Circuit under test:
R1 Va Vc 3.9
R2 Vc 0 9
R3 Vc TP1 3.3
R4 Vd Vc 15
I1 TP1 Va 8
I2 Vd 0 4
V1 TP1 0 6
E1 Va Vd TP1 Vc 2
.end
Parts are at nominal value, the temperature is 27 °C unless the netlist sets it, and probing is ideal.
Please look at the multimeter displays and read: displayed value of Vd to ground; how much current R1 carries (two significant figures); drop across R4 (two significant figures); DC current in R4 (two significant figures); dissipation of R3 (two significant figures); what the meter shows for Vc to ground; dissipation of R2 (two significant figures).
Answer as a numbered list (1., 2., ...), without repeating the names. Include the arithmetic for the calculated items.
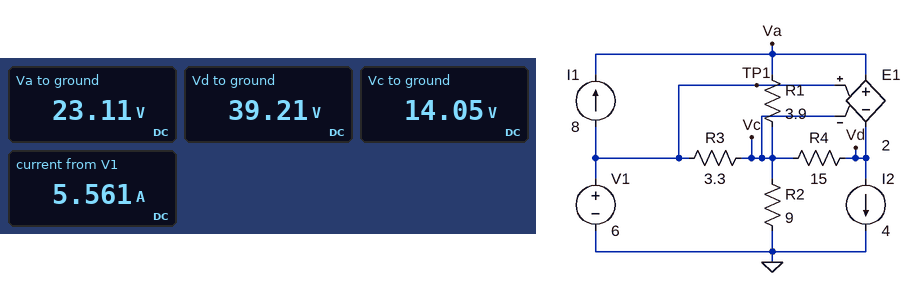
1. 39.21 V
2. (23.11 V - 14.05 V) / 3.9 Ω = 2.3 A
3. 39.21 V - 14.05 V = 25 V
4. (39.21 V - 14.05 V) / 15 Ω = 1.7 A
5. (14.05 V - 6 V)^2 / 3.3 Ω = 20 W
6. 14.05 V
7. (14.05 V)^2 / 9 Ω = 22 W
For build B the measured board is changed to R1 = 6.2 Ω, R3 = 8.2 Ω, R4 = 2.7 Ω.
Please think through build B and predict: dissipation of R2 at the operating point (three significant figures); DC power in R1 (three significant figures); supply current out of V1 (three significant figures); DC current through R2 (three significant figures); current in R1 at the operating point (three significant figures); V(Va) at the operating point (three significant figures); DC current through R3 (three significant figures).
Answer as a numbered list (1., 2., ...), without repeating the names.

1. 45.8 W
2. 24.8 W
3. 6.26 A
4. 2.26 A
5. 2.00 A
6. 7.90 V
7. 1.74 A
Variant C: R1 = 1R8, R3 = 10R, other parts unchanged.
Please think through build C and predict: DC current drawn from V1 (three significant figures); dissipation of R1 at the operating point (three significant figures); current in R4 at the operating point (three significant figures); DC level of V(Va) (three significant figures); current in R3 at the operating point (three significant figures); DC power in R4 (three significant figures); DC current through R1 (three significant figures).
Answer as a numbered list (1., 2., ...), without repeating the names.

1. 6.42 A
2. 5.15 W
3. 2.31 A
4. 24.8 V
5. 1.58 A
6. 79.9 W
7. 1.69 A
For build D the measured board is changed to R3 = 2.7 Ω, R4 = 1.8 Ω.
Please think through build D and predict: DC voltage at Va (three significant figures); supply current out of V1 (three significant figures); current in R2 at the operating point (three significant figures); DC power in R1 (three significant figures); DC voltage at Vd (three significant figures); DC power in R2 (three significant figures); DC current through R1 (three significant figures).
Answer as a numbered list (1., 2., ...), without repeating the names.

1. 8.38 V
2. 5.44 A
3. 1.44 A
4. 5.30 W
5. 22.2 V
6. 18.6 W
7. 1.17 A
